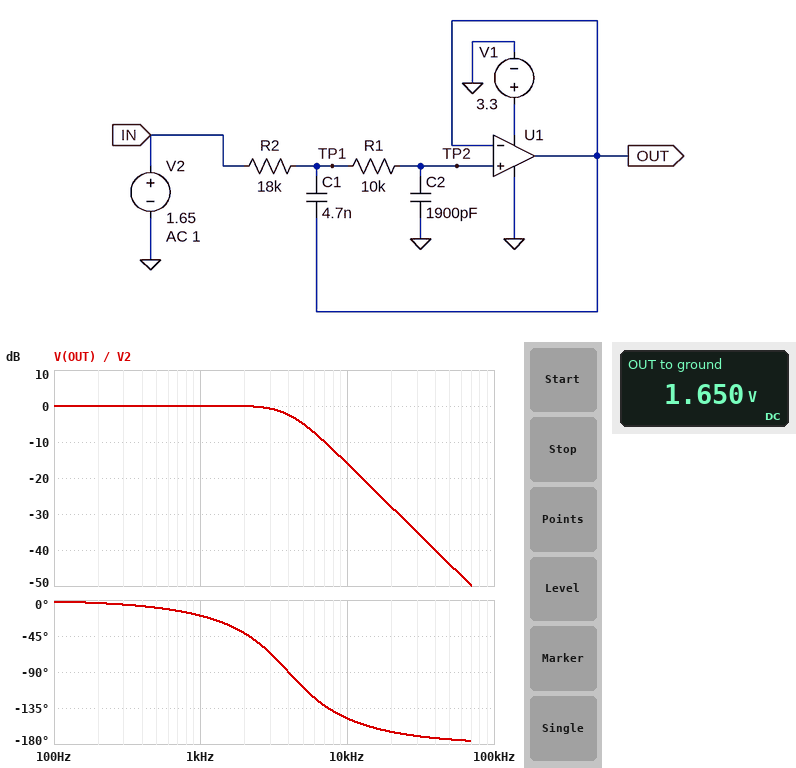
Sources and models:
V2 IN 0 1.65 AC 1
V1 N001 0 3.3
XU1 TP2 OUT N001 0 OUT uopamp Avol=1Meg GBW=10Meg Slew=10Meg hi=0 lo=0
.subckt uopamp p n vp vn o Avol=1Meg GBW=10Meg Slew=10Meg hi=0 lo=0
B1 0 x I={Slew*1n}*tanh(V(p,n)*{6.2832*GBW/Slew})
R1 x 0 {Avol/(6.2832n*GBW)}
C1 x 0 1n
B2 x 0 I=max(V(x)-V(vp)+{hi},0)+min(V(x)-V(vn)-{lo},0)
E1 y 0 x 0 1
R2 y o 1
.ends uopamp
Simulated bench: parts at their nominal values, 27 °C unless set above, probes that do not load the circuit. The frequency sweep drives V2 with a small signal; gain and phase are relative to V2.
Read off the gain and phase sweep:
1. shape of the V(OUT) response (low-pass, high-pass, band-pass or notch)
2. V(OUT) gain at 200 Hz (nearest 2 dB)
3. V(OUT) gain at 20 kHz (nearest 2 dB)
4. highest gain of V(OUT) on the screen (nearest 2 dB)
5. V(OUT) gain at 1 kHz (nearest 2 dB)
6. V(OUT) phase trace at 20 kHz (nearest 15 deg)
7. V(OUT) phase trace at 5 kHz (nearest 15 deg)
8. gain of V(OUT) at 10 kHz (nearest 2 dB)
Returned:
low-pass
0 dB
-28 dB
0 dB
0 dB
-165 deg
-105 deg
-16 dB
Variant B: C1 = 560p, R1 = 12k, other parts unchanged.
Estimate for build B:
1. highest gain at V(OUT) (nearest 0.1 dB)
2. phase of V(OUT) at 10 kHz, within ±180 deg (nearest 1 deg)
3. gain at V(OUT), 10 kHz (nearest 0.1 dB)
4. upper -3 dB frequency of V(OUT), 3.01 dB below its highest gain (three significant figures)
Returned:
0 dB
-89 deg
-11.1 dB
3.00 kHz
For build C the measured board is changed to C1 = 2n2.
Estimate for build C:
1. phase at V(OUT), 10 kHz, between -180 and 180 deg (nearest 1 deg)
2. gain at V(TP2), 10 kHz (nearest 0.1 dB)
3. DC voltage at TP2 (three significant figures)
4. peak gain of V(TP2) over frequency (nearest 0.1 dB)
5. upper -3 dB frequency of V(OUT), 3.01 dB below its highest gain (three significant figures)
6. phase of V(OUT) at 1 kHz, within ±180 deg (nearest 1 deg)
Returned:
-121 deg
-11.8 dB
1.65 V
0 dB
3.90 kHz
-19 deg
